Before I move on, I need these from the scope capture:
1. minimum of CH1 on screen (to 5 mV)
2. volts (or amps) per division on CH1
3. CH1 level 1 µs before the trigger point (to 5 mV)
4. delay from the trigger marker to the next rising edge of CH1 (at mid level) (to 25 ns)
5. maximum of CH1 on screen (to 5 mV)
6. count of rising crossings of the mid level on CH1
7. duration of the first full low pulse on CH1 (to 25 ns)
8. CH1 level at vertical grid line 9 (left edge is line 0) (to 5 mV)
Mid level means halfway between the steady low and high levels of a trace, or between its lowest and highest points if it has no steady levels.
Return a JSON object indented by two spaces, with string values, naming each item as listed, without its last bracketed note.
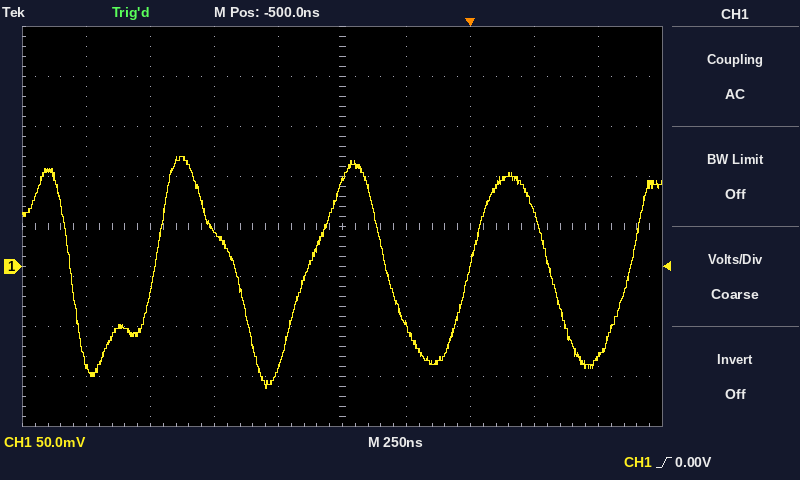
{
  "minimum of CH1 on screen": "-120 mV",
  "volts (or amps) per division on CH1": "50 mV",
  "CH1 level 1 µs before the trigger point": "35 mV",
  "delay from the trigger marker to the next rising edge of CH1 (at mid level)": "625 ns",
  "maximum of CH1 on screen": "110 mV",
  "count of rising crossings of the mid level on CH1": "4",
  "duration of the first full low pulse on CH1": "325 ns",
  "CH1 level at vertical grid line 9 (left edge is line 0)": "-90 mV"
}
